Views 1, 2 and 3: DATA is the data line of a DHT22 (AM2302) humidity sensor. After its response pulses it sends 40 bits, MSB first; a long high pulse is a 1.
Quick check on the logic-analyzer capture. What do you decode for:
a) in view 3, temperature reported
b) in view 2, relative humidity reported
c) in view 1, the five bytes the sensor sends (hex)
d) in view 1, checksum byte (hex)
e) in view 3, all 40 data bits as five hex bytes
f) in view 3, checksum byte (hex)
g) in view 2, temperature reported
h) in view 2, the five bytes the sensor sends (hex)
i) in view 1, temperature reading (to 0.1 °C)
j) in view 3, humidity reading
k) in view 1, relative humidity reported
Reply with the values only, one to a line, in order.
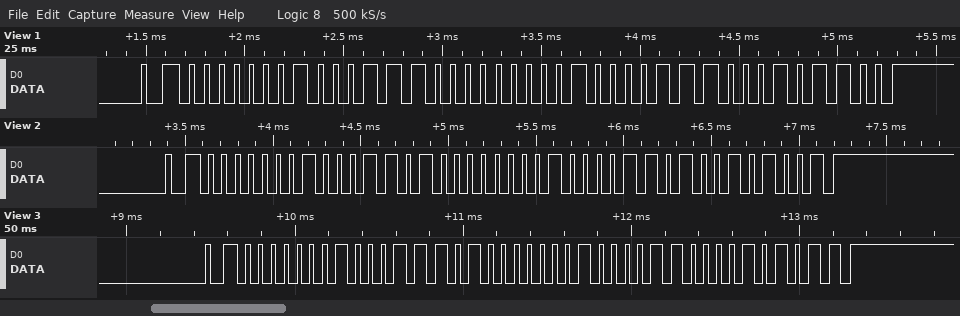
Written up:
26.8 °C
28.2 %
01 1C 01 0E 2C
0x2C
01 1D 01 0C 2B
0x2B
26.9 °C
01 1A 01 0D 29
27.0 °C
28.5 %
28.4 %
